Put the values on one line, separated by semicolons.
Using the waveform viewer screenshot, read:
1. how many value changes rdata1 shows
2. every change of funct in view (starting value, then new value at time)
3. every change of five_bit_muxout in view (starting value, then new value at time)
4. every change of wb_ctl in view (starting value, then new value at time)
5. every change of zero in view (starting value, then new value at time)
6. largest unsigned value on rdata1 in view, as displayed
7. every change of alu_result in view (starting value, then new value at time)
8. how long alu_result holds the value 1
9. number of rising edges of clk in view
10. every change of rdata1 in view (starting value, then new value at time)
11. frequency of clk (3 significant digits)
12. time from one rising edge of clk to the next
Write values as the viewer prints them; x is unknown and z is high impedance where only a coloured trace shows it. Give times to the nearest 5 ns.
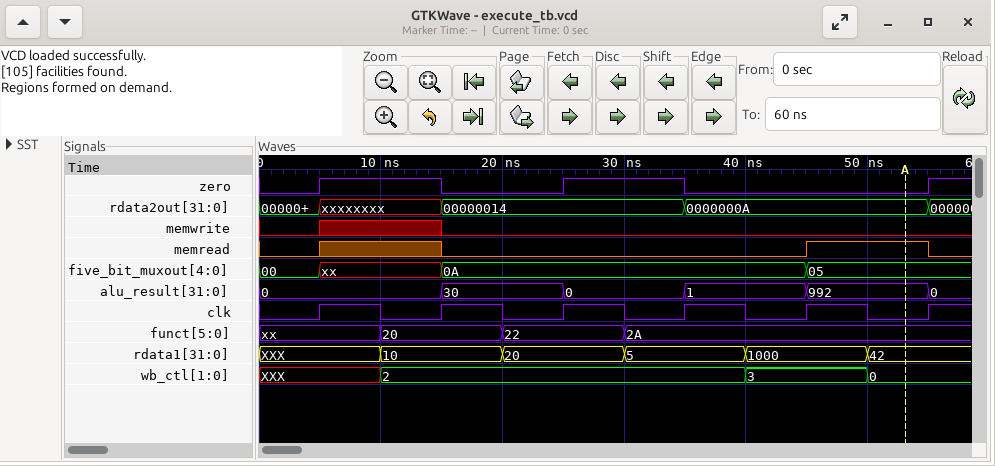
5; xx, 20 at 10 ns, 22 at 20 ns, 2A at 30 ns; 00, xx at 5 ns, 0A at 15 ns, 05 at 45 ns; XXX, 2 at 10 ns, 3 at 40 ns, 0 at 50 ns; 0, 1 at 5 ns, 0 at 15 ns, 1 at 25 ns, 0 at 35 ns, 1 at 55 ns; 1000; 0, 30 at 15 ns, 0 at 25 ns, 1 at 35 ns, 992 at 45 ns, 0 at 55 ns; 10 ns; 6; XXX, 10 at 10 ns, 20 at 20 ns, 5 at 30 ns, 1000 at 40 ns, 42 at 50 ns; 100 MHz; 10 ns
